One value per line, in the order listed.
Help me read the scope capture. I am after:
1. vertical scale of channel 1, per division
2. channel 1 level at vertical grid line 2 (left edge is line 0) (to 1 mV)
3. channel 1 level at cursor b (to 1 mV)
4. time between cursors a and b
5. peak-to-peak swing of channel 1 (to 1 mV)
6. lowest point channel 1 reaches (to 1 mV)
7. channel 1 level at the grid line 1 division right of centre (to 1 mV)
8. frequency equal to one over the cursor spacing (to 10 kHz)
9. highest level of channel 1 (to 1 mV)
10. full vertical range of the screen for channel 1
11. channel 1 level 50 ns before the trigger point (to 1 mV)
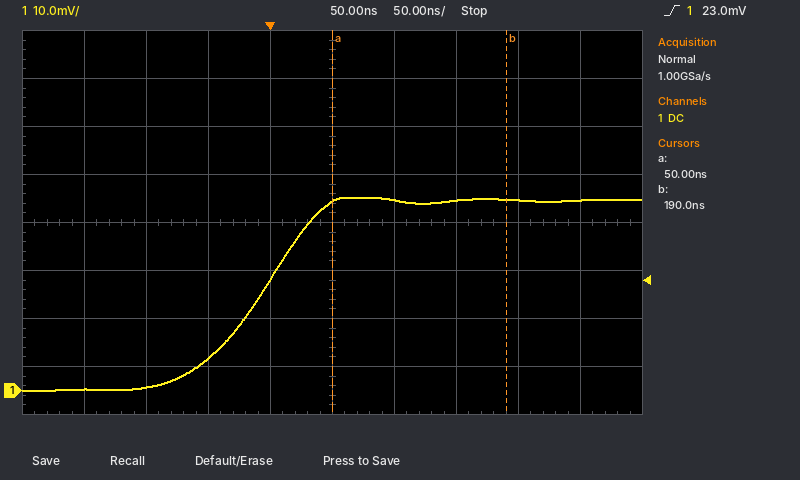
10 mV
1 mV
40 mV
140 ns
40 mV
0 mV
40 mV
7.14 MHz
40 mV
80 mV
7 mV
